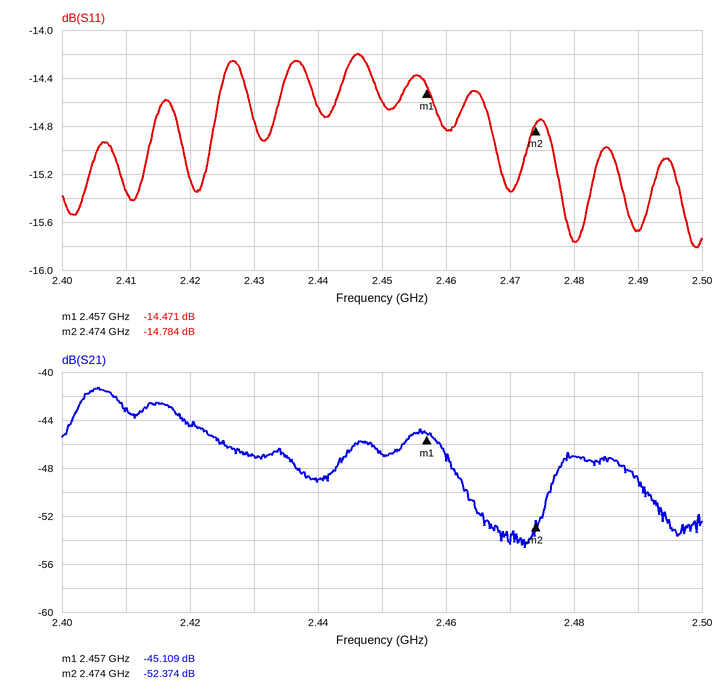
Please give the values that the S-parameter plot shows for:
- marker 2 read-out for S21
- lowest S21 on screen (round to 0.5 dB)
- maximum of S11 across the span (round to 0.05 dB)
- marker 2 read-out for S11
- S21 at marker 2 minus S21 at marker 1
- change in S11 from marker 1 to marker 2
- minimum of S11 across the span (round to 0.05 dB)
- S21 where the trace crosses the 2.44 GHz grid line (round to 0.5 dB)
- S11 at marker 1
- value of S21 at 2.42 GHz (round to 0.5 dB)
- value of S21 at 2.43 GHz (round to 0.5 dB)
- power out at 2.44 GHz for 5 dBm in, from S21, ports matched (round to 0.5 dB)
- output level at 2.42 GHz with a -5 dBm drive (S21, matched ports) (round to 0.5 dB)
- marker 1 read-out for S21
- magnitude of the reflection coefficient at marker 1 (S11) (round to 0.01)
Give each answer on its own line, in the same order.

-52.374 dB
-54.5 dB
-14.20 dB
-14.784 dB
-7.265 dB
-0.313 dB
-15.80 dB
-49.0 dB
-14.471 dB
-44.5 dB
-47.0 dB
-44.0 dBm
-49.5 dBm
-45.109 dB
0.19
